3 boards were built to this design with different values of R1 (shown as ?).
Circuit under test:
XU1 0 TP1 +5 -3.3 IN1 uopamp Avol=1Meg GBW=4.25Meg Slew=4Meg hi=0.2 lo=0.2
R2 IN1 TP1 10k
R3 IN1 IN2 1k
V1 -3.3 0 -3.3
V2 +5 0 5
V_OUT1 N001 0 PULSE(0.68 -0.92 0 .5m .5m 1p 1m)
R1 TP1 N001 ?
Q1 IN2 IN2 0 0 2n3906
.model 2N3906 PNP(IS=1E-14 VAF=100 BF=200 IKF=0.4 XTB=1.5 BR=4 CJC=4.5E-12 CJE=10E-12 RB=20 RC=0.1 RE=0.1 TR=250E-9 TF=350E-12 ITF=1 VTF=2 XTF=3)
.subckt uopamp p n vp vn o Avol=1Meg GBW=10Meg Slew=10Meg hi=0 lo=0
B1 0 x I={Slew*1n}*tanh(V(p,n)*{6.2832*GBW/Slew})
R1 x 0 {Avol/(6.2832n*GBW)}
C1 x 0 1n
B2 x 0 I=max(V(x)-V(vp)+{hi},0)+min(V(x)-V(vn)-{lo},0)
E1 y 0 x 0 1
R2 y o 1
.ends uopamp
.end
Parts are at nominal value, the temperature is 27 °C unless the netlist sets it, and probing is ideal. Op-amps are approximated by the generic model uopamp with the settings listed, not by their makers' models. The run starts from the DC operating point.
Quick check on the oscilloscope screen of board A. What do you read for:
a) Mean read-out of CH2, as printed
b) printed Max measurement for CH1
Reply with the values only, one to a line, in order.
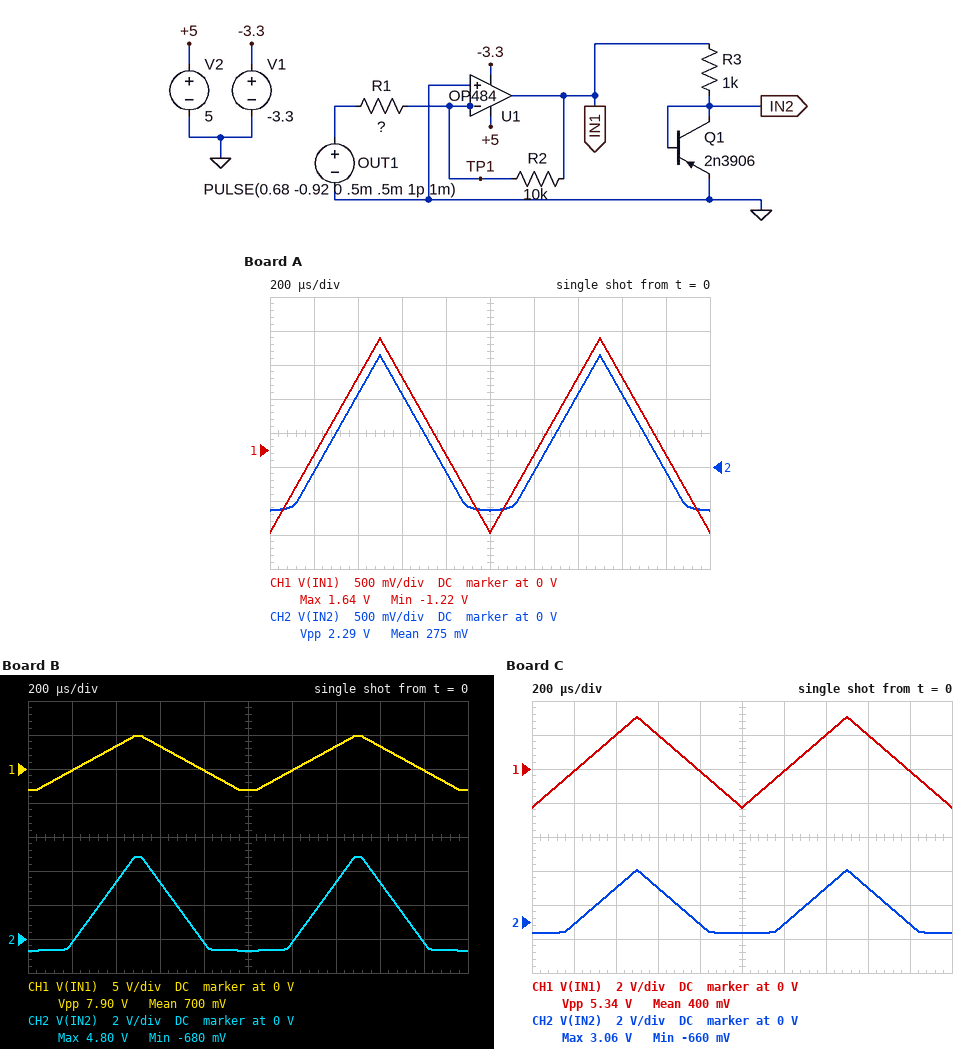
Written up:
275 mV
1.64 V
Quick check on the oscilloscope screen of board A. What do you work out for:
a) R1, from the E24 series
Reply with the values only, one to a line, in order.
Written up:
5.6 kΩ
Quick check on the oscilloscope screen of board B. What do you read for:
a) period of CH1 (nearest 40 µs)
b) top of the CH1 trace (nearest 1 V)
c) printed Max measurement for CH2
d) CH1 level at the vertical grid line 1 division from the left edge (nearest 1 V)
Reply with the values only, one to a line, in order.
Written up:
1.00 ms
5 V
4.80 V
0 V
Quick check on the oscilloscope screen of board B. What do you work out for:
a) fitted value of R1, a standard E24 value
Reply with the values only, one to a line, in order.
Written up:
1.8 kΩ
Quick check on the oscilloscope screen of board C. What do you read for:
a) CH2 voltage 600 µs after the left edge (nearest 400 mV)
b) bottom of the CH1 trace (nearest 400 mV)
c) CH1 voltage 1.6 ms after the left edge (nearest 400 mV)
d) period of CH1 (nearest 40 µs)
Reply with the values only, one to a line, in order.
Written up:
2.0 V
-2.4 V
2.0 V
1.00 ms
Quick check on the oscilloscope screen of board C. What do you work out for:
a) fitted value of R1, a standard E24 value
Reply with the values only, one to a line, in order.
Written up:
3 kΩ
